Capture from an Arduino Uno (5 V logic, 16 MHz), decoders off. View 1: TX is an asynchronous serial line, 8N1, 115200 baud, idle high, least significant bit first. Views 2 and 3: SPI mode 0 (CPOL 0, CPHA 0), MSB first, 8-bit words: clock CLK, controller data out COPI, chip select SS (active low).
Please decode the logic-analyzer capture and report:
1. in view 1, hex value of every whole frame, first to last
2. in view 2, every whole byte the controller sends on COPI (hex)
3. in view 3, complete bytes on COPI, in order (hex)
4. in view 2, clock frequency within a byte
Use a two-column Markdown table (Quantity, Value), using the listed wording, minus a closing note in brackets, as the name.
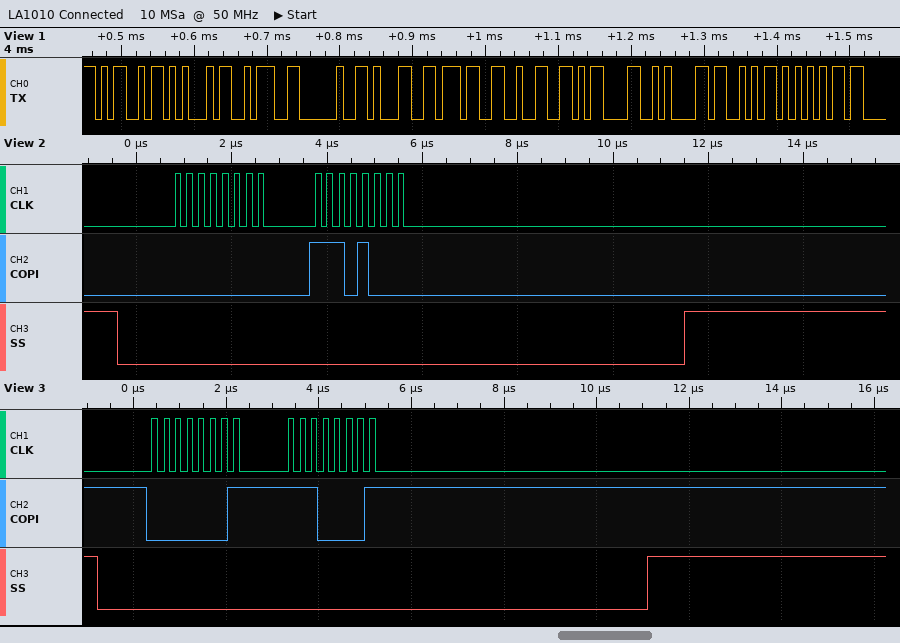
| Quantity | Value |
|---|---|
| in view 1, hex value of every whole frame, first to last | 0x4D 0x45 0x3A 0x20 0x31 0x37 0x32 0x0D 0x0A 0x53 0x55 |
| in view 2, every whole byte the controller sends on COPI | 00 E8 |
| in view 3, complete bytes on COPI, in order | 01 E1 |
| in view 2, clock frequency within a byte | 4 MHz |
